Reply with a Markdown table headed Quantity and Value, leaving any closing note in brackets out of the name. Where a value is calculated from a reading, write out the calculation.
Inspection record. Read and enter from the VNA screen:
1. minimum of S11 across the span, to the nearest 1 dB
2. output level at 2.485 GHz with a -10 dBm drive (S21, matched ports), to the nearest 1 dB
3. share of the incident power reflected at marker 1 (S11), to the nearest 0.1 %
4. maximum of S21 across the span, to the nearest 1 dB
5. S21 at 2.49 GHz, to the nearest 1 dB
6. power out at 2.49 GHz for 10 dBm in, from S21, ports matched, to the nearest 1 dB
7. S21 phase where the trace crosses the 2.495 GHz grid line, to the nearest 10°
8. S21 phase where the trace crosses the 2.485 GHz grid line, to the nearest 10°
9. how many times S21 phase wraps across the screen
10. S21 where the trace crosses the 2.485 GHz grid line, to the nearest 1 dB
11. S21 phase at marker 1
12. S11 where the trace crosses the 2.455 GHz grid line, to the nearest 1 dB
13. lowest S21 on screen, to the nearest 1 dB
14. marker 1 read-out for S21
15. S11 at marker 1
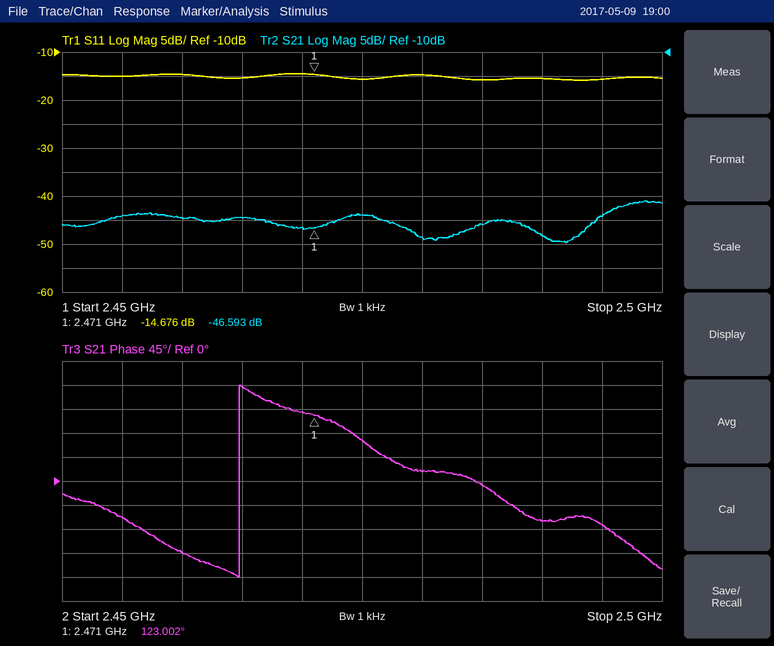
| Quantity | Value |
|---|---|
| minimum of S11 across the span, to the nearest 1 dB | -16 dB |
| output level at 2.485 GHz with a -10 dBm drive (S21, matched ports), to the nearest 1 dB | -10 dBm + (-46 dB) = -56 dBm |
| share of the incident power reflected at marker 1 (S11), to the nearest 0.1 % | 10^(-14.676/10) ≈ 3.4 % |
| maximum of S21 across the span, to the nearest 1 dB | -41 dB |
| S21 at 2.49 GHz, to the nearest 1 dB | -48 dB |
| power out at 2.49 GHz for 10 dBm in, from S21, ports matched, to the nearest 1 dB | 10 dBm + (-48 dB) = -38 dBm |
| S21 phase where the trace crosses the 2.495 GHz grid line, to the nearest 10° | -80° |
| S21 phase where the trace crosses the 2.485 GHz grid line, to the nearest 10° | -10° |
| how many times S21 phase wraps across the screen | 1 |
| S21 where the trace crosses the 2.485 GHz grid line, to the nearest 1 dB | -46 dB |
| S21 phase at marker 1 | 123.002° |
| S11 where the trace crosses the 2.455 GHz grid line, to the nearest 1 dB | -15 dB |
| lowest S21 on screen, to the nearest 1 dB | -50 dB |
| marker 1 read-out for S21 | -46.593 dB |
| S11 at marker 1 | -14.676 dB |
